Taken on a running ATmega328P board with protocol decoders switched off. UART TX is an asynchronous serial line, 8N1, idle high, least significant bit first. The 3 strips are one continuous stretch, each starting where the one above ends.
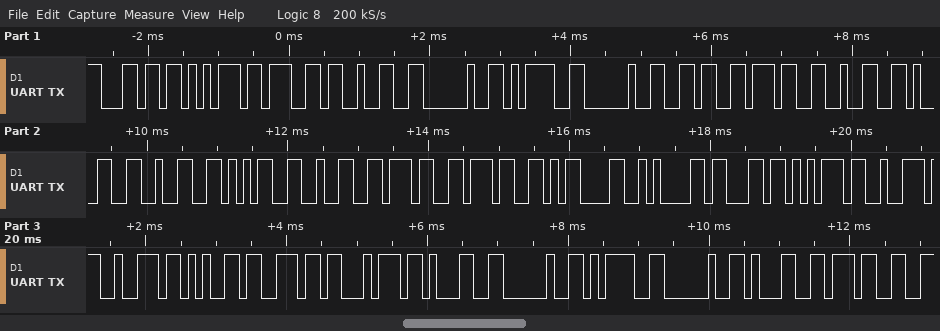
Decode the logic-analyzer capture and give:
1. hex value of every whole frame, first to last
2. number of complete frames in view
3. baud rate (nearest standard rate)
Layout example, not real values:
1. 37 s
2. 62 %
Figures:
1. 6C 75 67 32 20 3D 20 36 37 32 31 32 35 32 37 37 0D 0A 63 75 72 72 65 6E 74 31 20 3D 20 31 37
2. 31
3. 9600 baud
